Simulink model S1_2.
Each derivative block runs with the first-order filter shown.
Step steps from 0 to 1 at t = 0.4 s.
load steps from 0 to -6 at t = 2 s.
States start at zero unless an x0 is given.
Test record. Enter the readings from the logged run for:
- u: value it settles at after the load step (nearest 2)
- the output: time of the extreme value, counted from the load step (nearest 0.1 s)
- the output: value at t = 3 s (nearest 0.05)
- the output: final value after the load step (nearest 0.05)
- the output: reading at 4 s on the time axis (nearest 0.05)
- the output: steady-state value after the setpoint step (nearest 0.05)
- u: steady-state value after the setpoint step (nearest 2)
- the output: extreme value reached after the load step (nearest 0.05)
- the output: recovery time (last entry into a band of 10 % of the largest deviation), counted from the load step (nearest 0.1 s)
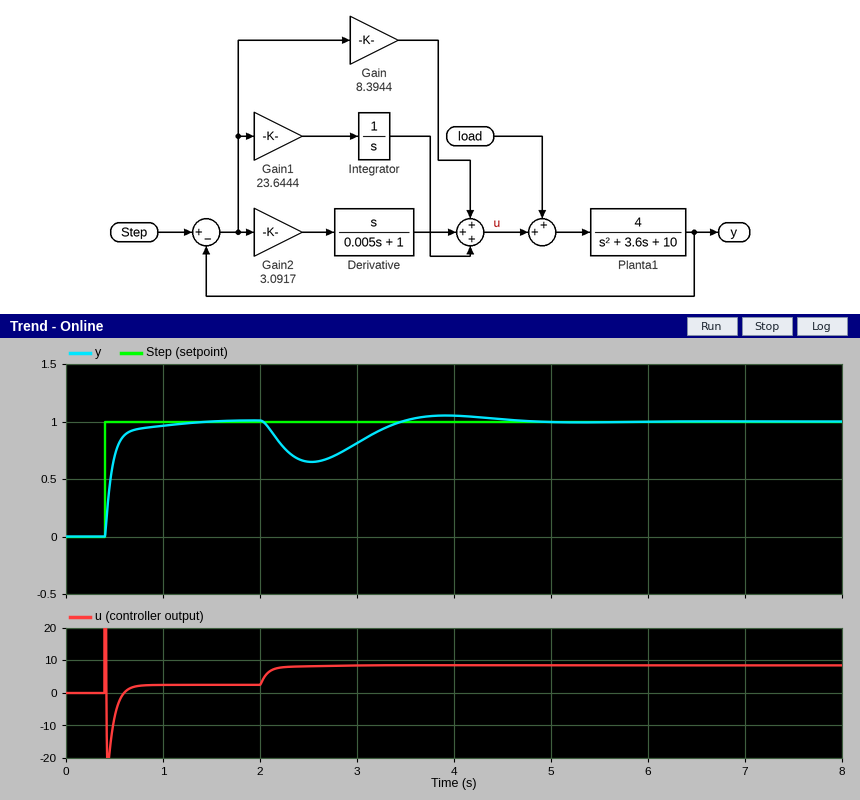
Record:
8
0.5 s
0.80
1.00
1.05
1.00
2
0.65
2.3 s
